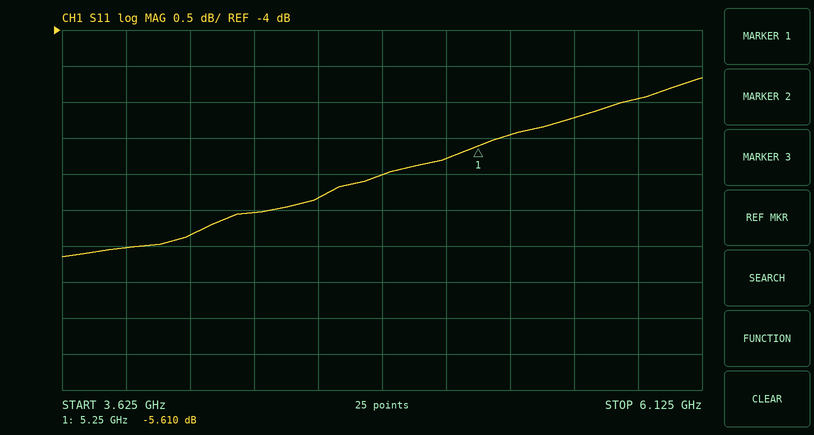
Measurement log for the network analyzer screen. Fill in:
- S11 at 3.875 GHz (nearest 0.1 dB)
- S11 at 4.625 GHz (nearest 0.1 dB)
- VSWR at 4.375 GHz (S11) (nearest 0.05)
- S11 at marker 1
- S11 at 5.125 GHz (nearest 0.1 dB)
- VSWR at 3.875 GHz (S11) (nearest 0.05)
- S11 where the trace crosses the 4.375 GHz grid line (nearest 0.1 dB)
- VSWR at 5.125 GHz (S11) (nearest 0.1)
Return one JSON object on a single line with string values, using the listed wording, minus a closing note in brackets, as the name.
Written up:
{"S11 at 3.875 GHz": "-7.0 dB", "S11 at 4.625 GHz": "-6.3 dB", "VSWR at 4.375 GHz (S11)": "2.80", "S11 at marker 1": "-5.610 dB", "S11 at 5.125 GHz": "-5.8 dB", "VSWR at 3.875 GHz (S11)": "2.60", "S11 where the trace crosses the 4.375 GHz grid line": "-6.5 dB", "VSWR at 5.125 GHz (S11)": "3.1"}
